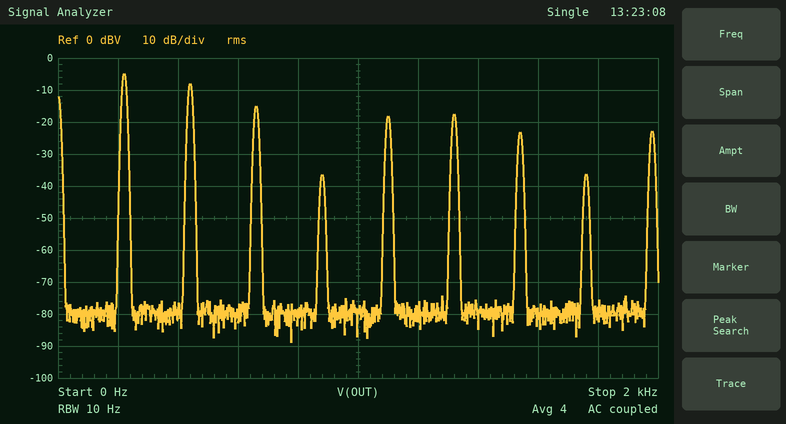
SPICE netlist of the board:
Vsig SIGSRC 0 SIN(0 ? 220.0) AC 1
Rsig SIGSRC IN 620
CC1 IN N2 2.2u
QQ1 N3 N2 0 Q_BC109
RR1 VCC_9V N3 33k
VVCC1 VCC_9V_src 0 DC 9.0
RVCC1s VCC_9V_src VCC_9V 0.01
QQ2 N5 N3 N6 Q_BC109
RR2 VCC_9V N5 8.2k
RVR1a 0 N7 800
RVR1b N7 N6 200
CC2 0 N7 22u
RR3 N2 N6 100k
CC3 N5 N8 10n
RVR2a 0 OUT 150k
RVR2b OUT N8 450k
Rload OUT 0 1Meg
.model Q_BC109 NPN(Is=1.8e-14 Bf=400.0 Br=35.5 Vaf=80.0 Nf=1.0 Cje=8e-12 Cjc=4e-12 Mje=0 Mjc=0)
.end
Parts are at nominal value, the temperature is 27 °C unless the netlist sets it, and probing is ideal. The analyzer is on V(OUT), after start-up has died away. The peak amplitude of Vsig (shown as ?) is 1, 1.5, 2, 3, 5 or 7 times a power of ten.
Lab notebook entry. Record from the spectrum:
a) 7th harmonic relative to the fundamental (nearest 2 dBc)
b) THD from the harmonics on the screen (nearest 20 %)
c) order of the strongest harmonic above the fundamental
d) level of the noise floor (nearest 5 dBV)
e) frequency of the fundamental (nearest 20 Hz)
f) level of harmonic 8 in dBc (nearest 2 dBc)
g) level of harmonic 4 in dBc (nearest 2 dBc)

-18 dBc
80 %
2
-80 dBV
220 Hz
-32 dBc
-32 dBc
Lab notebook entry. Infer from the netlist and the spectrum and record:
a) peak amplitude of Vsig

200 mV
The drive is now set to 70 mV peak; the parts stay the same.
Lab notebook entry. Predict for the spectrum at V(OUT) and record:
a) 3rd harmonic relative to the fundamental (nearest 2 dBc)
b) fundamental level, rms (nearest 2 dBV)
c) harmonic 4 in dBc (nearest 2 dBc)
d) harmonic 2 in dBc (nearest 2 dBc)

-32 dBc
-4 dBV
-12 dBc
-6 dBc
